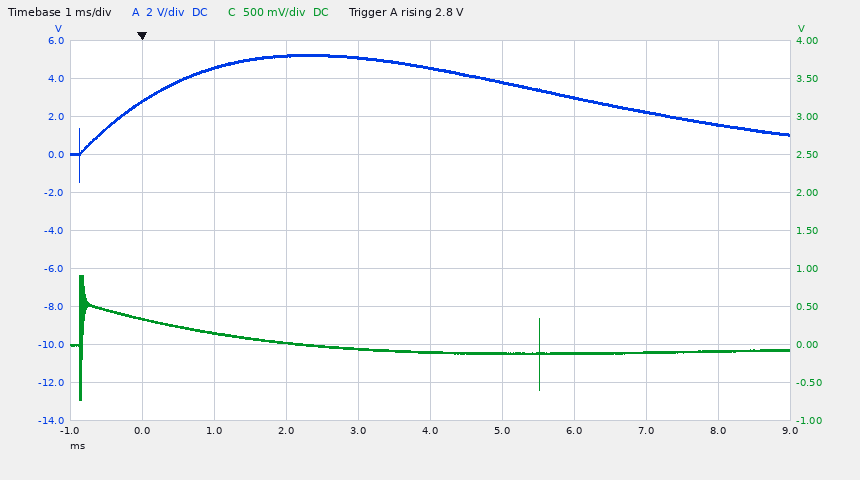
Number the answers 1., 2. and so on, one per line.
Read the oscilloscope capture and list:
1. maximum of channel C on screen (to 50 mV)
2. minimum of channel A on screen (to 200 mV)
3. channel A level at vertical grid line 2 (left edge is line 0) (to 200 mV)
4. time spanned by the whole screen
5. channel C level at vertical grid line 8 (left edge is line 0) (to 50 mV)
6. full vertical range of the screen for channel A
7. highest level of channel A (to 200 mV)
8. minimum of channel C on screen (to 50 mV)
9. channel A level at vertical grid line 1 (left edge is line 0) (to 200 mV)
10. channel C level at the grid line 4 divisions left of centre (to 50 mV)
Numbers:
1. 900 mV
2. -1.4 V
3. 4.6 V
4. 10 ms
5. -100 mV
6. 20 V
7. 5.2 V
8. -700 mV
9. 2.8 V
10. 350 mV
